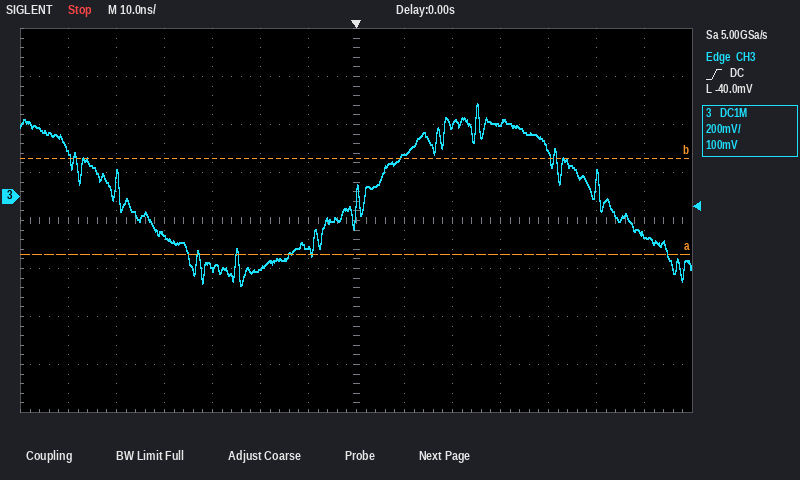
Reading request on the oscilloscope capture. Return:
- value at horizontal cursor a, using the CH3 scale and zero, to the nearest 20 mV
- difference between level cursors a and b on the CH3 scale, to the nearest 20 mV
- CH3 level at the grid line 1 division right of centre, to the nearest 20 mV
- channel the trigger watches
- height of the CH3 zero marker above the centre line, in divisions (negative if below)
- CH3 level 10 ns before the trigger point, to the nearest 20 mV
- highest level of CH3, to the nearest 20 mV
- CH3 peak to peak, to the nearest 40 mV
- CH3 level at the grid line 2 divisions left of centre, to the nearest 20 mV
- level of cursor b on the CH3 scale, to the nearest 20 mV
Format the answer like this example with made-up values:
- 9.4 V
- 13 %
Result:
- -240 mV
- 400 mV
- 180 mV
- CH3
- +0.5 div
- -220 mV
- 380 mV
- 760 mV
- -300 mV
- 160 mV
